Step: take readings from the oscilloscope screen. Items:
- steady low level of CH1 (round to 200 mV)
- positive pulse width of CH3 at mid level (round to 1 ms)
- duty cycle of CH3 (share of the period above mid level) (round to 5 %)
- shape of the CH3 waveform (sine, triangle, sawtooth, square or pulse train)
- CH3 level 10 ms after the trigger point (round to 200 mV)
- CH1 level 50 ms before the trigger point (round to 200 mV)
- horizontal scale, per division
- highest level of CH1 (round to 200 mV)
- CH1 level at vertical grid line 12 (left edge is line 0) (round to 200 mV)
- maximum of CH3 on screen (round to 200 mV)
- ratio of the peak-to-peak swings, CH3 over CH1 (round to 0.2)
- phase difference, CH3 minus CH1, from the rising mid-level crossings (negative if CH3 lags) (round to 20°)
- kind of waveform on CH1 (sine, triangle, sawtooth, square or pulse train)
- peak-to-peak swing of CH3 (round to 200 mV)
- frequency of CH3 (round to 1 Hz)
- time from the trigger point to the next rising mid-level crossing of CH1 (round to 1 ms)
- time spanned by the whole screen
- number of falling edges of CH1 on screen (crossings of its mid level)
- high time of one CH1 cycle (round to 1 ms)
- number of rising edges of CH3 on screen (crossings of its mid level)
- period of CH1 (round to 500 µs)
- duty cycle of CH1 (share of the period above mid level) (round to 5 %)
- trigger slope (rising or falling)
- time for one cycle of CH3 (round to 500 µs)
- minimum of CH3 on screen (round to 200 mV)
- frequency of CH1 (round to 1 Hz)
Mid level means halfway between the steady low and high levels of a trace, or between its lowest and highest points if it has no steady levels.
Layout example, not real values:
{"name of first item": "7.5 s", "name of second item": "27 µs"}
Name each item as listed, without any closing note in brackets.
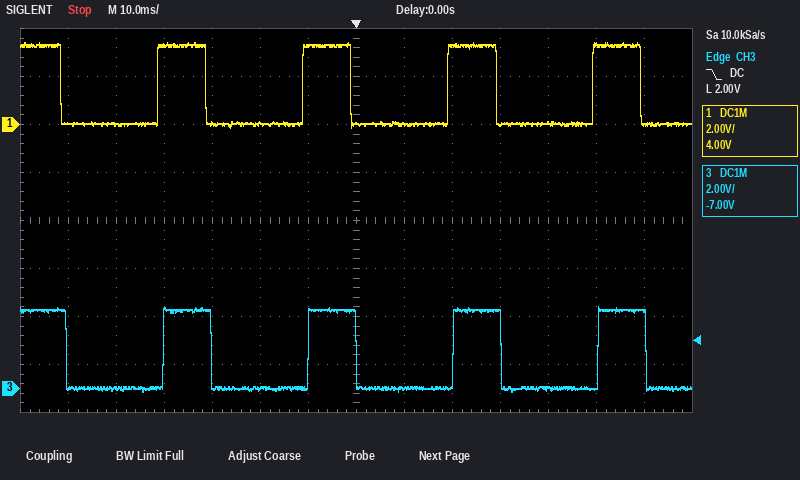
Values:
{"steady low level of CH1": "0.0 V", "positive pulse width of CH3 at mid level": "10 ms", "duty cycle of CH3 (share of the period above mid level)": "35 %", "shape of the CH3 waveform": "pulse train", "CH3 level 10 ms after the trigger point": "0.0 V", "CH1 level 50 ms before the trigger point": "0.0 V", "horizontal scale, per division": "10 ms", "highest level of CH1": "3.4 V", "CH1 level at vertical grid line 12 (left edge is line 0)": "3.4 V", "maximum of CH3 on screen": "3.4 V", "ratio of the peak-to-peak swings, CH3 over CH1": "1.0", "phase difference, CH3 minus CH1, from the rising mid-level crossings (negative if CH3 lags)": "-20°", "kind of waveform on CH1": "pulse train", "peak-to-peak swing of CH3": "3.6 V", "frequency of CH3": "33 Hz", "time from the trigger point to the next rising mid-level crossing of CH1": "19 ms", "time spanned by the whole screen": "140 ms", "number of falling edges of CH1 on screen": "5", "high time of one CH1 cycle": "10 ms", "number of rising edges of CH3 on screen": "4", "period of CH1": "30.0 ms", "duty cycle of CH1 (share of the period above mid level)": "35 %", "trigger slope": "falling", "time for one cycle of CH3": "30.0 ms", "minimum of CH3 on screen": "-200 mV", "frequency of CH1": "33 Hz"}
